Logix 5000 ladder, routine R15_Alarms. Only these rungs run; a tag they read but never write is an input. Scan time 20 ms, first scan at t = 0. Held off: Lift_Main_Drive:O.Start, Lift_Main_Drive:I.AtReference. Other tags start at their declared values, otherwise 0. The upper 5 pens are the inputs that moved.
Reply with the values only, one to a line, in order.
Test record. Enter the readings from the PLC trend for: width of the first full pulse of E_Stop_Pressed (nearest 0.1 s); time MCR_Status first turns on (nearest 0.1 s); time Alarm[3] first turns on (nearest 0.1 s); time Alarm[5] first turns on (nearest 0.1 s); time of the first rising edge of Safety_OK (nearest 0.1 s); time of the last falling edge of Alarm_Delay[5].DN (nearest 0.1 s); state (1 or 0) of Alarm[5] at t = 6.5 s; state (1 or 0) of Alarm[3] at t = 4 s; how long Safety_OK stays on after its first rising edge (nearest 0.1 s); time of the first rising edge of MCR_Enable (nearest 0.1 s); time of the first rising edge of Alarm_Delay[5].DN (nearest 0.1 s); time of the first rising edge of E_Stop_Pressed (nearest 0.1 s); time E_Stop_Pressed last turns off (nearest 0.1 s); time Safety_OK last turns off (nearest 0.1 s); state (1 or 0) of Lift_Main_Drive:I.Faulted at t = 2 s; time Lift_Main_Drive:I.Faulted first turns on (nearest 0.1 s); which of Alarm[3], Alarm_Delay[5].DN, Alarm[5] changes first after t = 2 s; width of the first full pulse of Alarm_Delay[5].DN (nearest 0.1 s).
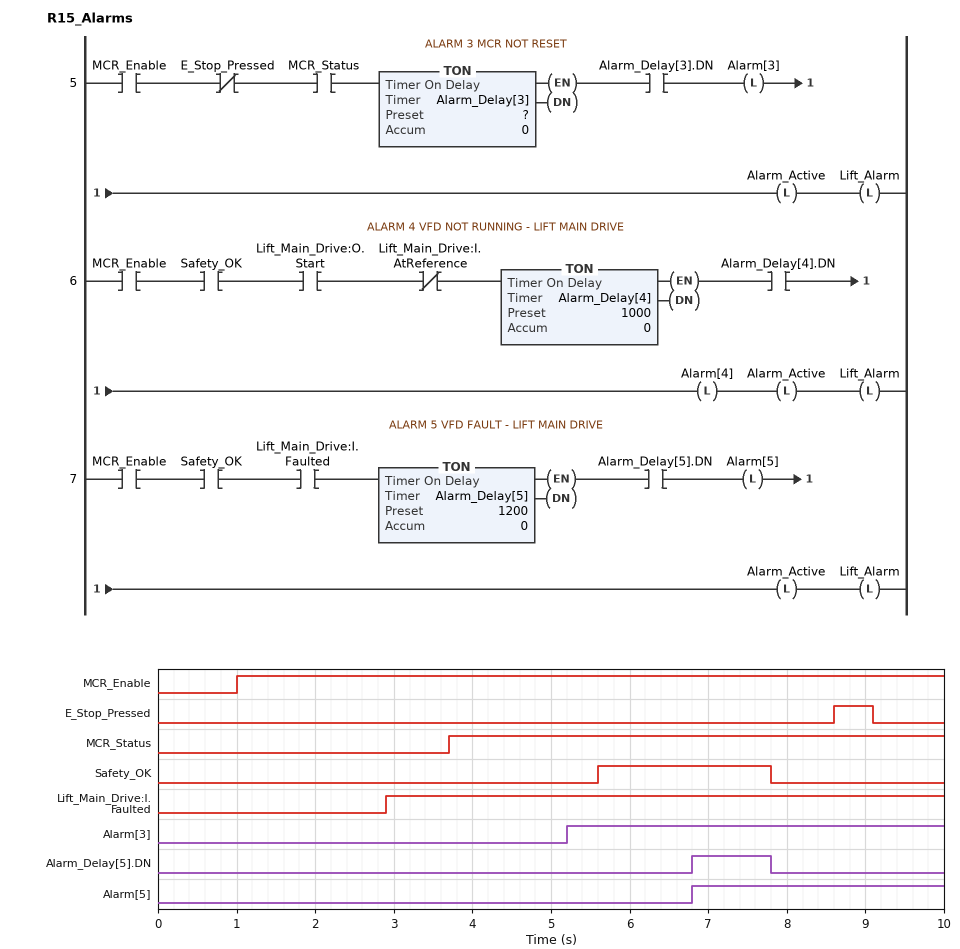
0.5 s
3.7 s
5.2 s
6.8 s
5.6 s
7.8 s
0
0
2.2 s
1.0 s
6.8 s
8.6 s
9.1 s
7.8 s
0
2.9 s
Alarm[3]
1.0 s
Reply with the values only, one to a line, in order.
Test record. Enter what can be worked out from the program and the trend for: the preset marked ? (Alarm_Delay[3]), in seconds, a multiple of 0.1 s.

1.5 s
